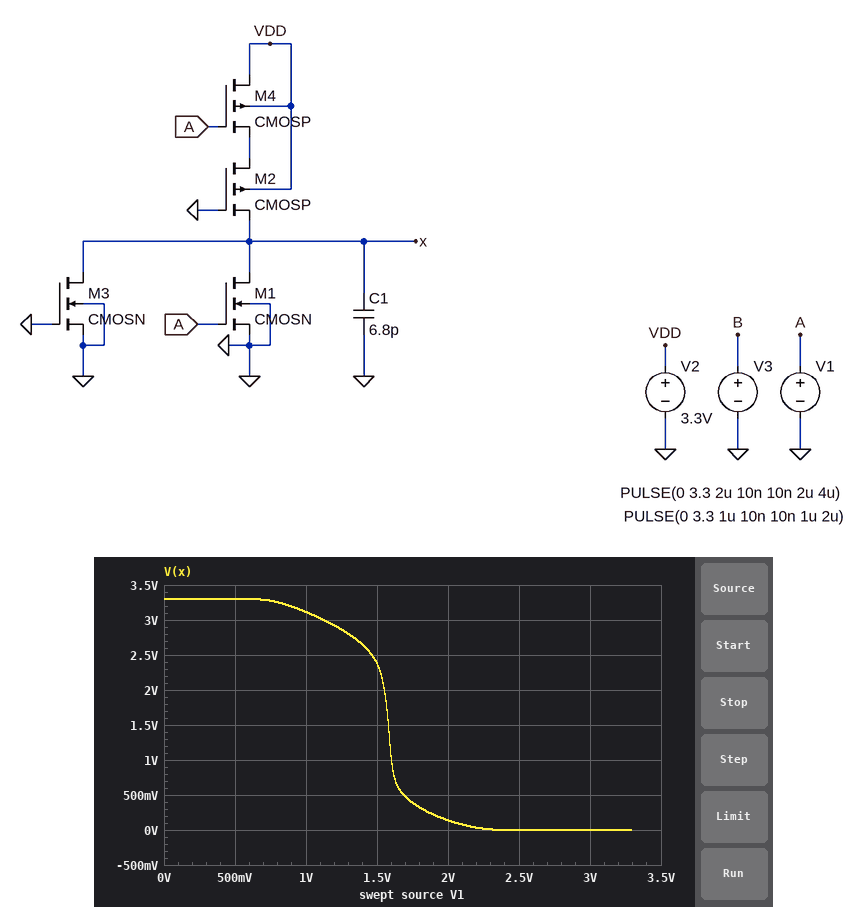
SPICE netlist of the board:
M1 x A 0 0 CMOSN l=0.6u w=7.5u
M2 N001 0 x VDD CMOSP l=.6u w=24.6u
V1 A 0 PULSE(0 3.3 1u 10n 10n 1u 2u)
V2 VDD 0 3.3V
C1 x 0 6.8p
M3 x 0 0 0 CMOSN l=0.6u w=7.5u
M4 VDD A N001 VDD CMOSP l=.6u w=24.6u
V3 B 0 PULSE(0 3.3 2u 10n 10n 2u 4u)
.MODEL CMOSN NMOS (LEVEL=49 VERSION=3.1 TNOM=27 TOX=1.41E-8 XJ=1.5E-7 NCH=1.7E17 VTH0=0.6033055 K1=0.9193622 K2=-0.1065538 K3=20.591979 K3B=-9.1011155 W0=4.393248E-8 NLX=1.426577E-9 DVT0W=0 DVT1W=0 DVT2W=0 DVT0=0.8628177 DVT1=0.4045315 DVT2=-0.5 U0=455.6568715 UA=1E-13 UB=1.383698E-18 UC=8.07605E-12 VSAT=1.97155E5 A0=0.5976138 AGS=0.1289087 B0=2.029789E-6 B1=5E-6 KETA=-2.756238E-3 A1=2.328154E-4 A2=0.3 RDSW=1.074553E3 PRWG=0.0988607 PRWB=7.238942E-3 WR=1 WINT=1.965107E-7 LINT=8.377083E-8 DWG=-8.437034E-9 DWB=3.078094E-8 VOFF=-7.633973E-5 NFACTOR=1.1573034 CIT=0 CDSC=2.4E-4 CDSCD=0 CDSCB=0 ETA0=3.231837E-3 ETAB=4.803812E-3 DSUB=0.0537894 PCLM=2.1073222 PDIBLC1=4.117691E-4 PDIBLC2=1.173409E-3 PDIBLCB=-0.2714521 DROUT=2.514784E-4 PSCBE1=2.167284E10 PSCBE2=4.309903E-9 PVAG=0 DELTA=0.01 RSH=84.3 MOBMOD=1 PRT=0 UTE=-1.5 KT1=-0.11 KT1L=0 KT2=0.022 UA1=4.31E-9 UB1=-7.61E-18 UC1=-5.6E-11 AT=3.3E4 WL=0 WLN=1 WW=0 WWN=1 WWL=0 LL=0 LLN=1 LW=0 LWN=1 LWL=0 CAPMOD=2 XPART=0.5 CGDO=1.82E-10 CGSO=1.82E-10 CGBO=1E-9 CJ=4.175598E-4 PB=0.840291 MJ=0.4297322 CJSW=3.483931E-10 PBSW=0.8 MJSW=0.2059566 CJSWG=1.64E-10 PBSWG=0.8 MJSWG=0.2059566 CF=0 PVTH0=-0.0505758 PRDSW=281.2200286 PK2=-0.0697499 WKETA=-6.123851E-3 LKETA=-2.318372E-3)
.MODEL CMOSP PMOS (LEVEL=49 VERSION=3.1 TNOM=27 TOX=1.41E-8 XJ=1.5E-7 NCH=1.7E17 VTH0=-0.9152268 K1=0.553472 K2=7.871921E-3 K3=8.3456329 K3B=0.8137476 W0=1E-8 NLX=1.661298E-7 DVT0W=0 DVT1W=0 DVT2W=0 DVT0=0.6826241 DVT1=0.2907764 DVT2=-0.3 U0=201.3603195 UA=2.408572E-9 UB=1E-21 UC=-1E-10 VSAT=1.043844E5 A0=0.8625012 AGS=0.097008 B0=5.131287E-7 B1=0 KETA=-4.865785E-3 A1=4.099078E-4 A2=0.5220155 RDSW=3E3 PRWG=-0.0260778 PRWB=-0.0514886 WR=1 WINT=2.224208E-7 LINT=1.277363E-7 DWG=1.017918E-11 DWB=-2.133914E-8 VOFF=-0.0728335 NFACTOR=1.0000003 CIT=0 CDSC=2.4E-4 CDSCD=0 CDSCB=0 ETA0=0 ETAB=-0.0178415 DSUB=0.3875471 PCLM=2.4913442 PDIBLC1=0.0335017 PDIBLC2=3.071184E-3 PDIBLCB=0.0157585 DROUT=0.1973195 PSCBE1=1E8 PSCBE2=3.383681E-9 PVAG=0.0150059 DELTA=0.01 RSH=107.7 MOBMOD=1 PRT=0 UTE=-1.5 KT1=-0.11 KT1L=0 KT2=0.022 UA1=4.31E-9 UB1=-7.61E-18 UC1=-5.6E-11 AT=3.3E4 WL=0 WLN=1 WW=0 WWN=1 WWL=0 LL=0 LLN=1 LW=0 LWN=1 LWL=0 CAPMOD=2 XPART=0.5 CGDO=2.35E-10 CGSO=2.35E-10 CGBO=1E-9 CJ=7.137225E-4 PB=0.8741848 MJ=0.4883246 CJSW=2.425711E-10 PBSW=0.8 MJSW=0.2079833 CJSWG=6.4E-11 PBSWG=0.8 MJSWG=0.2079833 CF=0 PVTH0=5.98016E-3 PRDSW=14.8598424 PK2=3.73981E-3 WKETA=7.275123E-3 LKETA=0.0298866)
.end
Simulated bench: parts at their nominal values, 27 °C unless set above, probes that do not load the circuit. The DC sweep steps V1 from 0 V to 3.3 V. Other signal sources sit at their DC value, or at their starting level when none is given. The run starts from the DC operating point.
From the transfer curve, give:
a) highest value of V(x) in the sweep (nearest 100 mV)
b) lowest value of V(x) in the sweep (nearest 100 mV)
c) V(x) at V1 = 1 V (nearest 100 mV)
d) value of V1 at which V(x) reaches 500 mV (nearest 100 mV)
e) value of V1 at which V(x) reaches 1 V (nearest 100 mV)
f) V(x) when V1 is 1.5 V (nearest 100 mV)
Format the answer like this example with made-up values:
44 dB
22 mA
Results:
3.3 V
0 V
3.1 V
1.7 V
1.6 V
2.4 V
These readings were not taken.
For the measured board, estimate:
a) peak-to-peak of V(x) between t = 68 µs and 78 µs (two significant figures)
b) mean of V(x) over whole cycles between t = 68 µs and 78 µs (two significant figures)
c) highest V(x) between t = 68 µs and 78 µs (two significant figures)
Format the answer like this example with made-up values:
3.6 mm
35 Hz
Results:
3.3 V
1.6 V
3.3 V
